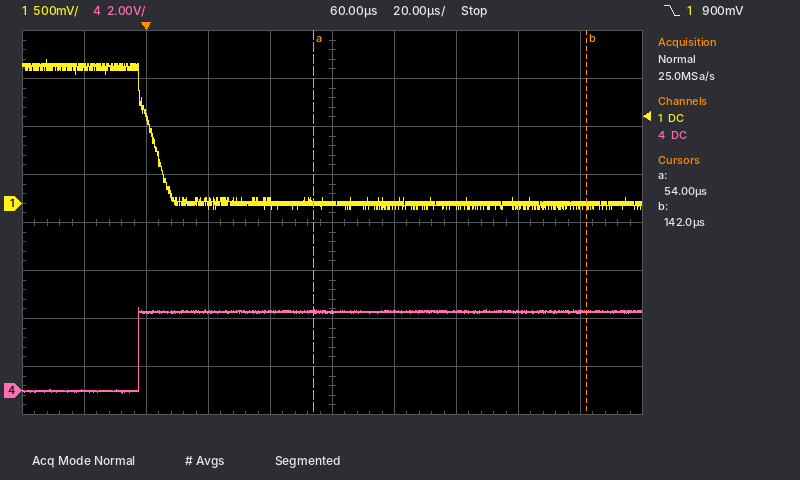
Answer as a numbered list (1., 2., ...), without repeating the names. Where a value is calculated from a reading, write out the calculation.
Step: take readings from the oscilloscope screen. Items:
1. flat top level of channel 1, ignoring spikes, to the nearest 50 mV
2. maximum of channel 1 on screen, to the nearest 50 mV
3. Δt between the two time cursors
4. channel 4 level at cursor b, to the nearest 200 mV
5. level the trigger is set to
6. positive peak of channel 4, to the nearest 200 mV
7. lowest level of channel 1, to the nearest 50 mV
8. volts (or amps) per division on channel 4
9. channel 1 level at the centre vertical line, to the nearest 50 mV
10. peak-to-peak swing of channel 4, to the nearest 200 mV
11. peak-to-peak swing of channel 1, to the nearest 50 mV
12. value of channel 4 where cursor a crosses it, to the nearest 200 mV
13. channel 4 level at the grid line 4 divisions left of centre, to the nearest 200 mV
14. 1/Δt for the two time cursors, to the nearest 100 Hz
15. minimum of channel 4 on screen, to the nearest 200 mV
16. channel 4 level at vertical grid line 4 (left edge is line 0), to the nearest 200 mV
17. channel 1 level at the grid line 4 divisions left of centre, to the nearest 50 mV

1. 1.40 V
2. 1.50 V
3. 142 µs − (54 µs) = 88 µs
4. 3.2 V
5. 900 mV
6. 3.4 V
7. -50 mV
8. 2 V
9. 0 mV
10. 3.4 V − (-200 mV) = 3.6 V
11. 1.50 V − (-50 mV) = 1.55 V
12. 3.2 V
13. 0.0 V
14. 1 / 88 µs ≈ 11.4 kHz
15. -200 mV
16. 3.2 V
17. 1.40 V
